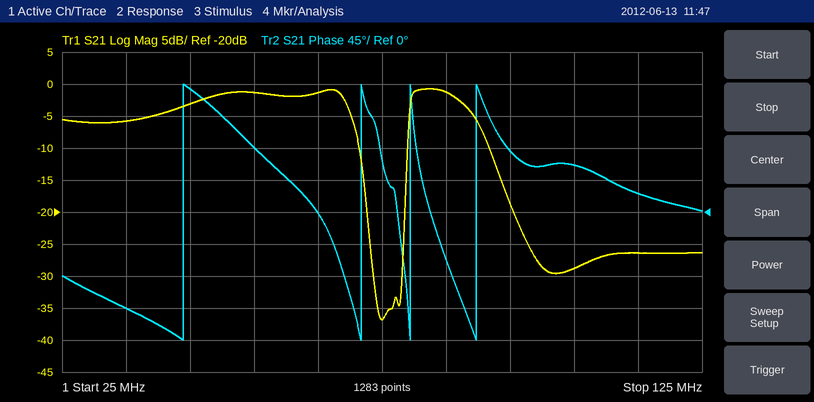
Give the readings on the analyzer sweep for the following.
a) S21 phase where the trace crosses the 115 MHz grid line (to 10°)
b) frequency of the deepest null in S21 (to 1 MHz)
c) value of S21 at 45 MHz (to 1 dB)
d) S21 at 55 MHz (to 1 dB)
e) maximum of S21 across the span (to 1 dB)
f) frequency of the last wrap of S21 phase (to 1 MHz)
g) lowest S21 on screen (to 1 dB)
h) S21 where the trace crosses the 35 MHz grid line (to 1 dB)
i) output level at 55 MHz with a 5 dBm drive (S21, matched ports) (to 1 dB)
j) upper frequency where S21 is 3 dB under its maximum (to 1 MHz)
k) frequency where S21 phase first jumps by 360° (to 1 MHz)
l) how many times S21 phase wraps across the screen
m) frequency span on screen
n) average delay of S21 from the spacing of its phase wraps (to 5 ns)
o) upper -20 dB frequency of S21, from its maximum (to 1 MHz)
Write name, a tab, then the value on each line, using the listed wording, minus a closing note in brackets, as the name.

S21 phase where the trace crosses the 115 MHz grid line	30°
frequency of the deepest null in S21	75 MHz
value of S21 at 45 MHz	-3 dB
S21 at 55 MHz	-1 dB
maximum of S21 across the span	-1 dB
frequency of the last wrap of S21 phase	90 MHz
lowest S21 on screen	-37 dB
S21 where the trace crosses the 35 MHz grid line	-6 dB
output level at 55 MHz with a 5 dBm drive (S21, matched ports)	4 dBm
upper frequency where S21 is 3 dB under its maximum	88 MHz
frequency where S21 phase first jumps by 360°	44 MHz
how many times S21 phase wraps across the screen	4
frequency span on screen	100 MHz
average delay of S21 from the spacing of its phase wraps	65 ns
upper -20 dB frequency of S21, from its maximum	96 MHz
